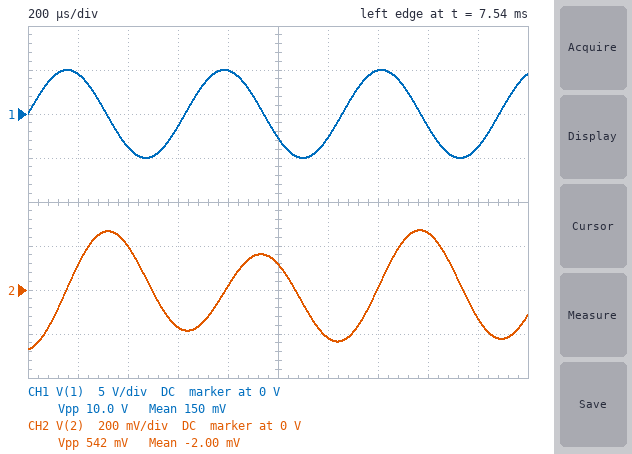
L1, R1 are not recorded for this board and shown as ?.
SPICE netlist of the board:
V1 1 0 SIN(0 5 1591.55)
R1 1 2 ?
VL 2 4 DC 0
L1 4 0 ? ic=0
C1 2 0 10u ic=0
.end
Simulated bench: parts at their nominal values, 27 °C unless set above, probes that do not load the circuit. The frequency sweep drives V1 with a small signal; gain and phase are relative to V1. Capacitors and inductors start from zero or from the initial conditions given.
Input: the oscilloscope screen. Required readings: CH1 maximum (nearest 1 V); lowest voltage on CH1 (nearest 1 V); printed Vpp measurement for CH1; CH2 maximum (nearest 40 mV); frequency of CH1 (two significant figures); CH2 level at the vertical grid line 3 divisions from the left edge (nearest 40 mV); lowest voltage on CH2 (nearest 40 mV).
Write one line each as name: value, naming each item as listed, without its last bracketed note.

CH1 maximum: 5 V
lowest voltage on CH1: -5 V
printed Vpp measurement for CH1: 10.0 V
CH2 maximum: 280 mV
frequency of CH1: 1.6 kHz
CH2 level at the vertical grid line 3 divisions from the left edge: -160 mV
lowest voltage on CH2: -280 mV
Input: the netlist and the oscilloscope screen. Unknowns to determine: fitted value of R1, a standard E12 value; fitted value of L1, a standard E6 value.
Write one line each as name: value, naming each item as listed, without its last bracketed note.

fitted value of R1, a standard E12 value: 330 Ω
fitted value of L1, a standard E6 value: 3.3 mH
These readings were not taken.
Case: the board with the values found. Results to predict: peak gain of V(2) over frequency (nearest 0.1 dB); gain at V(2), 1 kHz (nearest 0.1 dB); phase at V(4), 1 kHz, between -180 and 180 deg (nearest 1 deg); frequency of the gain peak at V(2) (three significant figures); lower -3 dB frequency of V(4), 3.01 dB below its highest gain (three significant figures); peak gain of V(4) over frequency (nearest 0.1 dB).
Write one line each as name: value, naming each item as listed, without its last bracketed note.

peak gain of V(2) over frequency: 0 dB
gain at V(2), 1 kHz: -13.8 dB
phase at V(4), 1 kHz, between -180 and 180 deg: -78 deg
frequency of the gain peak at V(2): 876 Hz
lower -3 dB frequency of V(4), 3.01 dB below its highest gain: 852 Hz
peak gain of V(4) over frequency: 0 dB
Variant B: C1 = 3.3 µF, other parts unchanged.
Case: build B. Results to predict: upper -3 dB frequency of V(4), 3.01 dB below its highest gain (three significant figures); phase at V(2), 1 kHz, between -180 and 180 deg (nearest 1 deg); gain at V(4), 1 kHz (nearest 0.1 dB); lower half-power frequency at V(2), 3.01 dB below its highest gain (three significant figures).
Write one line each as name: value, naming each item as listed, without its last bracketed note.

upper -3 dB frequency of V(4), 3.01 dB below its highest gain: 1.60 kHz
phase at V(2), 1 kHz, between -180 and 180 deg: 84 deg
gain at V(4), 1 kHz: -19.2 dB
lower half-power frequency at V(2), 3.01 dB below its highest gain: 1.45 kHz
